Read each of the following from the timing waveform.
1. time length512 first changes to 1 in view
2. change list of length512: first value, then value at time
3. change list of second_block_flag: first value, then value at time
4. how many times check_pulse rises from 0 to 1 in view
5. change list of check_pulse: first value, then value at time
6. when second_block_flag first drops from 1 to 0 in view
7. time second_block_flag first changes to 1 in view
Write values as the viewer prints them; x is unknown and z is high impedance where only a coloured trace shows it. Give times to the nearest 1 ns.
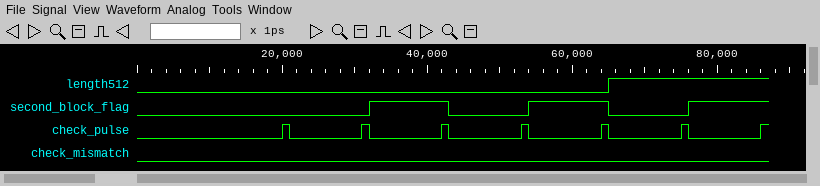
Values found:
65 ns
0, 1 at 65 ns
0, 1 at 32 ns, 0 at 43 ns, 1 at 54 ns, 0 at 65 ns, 1 at 76 ns
7
0, 1 at 20 ns, 0 at 21 ns, 1 at 31 ns, 0 at 32 ns, 1 at 42 ns, 0 at 43 ns, 1 at 53 ns, 0 at 54 ns, 1 at 64 ns, 0 at 65 ns, 1 at 75 ns, 0 at 76 ns, 1 at 86 ns
43 ns
32 ns
